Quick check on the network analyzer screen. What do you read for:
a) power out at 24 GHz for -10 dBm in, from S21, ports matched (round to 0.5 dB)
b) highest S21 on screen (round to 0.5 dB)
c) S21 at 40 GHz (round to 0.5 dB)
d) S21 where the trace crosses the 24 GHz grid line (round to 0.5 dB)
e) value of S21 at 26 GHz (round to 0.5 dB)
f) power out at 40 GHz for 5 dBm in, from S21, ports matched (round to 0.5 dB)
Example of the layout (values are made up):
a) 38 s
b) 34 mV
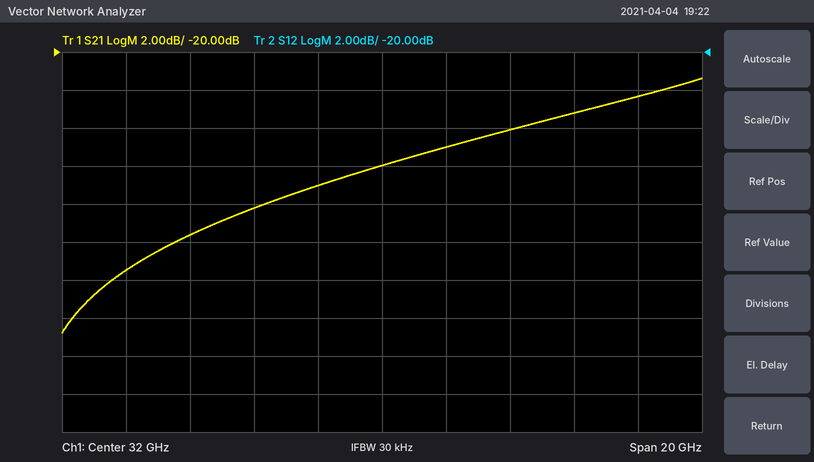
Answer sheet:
a) -41.5 dBm
b) -21.5 dB
c) -22.5 dB
d) -31.5 dB
e) -29.5 dB
f) -17.5 dBm
